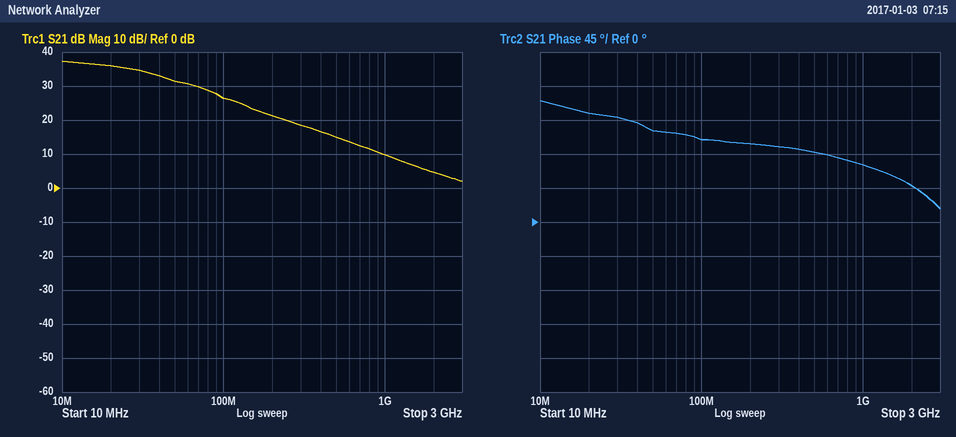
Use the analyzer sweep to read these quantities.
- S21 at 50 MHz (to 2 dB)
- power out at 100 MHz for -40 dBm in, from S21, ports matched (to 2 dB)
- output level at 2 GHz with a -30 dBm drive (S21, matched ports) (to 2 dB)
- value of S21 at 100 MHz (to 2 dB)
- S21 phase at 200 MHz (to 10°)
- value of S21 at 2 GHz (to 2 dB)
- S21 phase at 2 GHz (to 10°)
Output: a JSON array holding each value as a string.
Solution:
["32 dB", "-14 dBm", "-26 dBm", "26 dB", "100°", "4 dB", "50°"]
